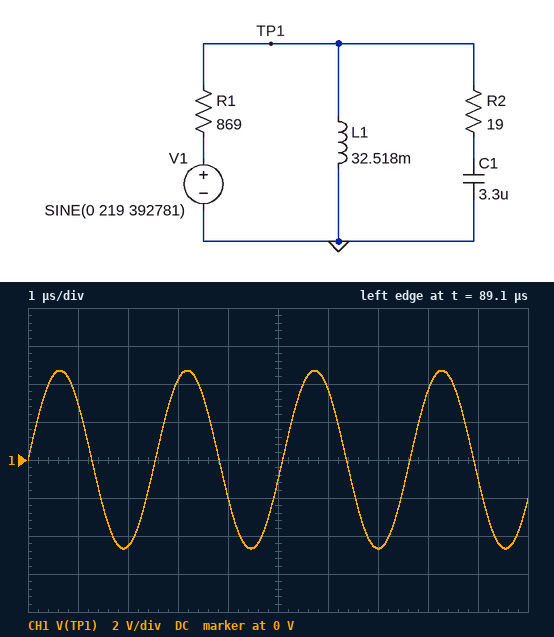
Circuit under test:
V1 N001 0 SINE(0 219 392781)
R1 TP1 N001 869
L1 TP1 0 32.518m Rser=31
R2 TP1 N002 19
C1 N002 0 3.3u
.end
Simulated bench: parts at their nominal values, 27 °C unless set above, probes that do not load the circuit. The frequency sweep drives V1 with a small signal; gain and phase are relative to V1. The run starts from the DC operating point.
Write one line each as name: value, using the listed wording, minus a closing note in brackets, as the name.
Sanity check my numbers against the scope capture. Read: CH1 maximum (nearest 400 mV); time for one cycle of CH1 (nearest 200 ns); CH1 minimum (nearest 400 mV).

CH1 maximum: 4.8 V
time for one cycle of CH1: 2.6 µs
CH1 minimum: -4.8 V
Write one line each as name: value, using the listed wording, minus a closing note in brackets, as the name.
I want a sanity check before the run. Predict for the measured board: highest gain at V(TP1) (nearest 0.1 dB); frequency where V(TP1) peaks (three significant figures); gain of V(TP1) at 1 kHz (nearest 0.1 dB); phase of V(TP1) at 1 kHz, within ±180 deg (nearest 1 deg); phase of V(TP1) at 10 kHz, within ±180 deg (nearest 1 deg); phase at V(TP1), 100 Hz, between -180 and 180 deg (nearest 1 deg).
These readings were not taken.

highest gain at V(TP1): -14.2 dB
frequency where V(TP1) peaks: 487 Hz
gain of V(TP1) at 1 kHz: -22.8 dB
phase of V(TP1) at 1 kHz, within ±180 deg: -56 deg
phase of V(TP1) at 10 kHz, within ±180 deg: -13 deg
phase at V(TP1), 100 Hz, between -180 and 180 deg: 28 deg
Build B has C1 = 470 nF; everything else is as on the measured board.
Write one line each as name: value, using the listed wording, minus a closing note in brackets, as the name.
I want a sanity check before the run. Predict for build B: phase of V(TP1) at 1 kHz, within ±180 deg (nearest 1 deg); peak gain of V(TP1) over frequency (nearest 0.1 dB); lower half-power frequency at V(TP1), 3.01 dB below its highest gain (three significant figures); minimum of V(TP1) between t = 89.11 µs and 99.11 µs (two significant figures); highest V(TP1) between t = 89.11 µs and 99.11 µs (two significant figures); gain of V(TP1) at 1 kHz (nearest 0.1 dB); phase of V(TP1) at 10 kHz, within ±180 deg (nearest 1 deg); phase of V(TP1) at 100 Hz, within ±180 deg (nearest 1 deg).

phase of V(TP1) at 1 kHz, within ±180 deg: 42 deg
peak gain of V(TP1) over frequency: -4.2 dB
lower half-power frequency at V(TP1), 3.01 dB below its highest gain: 1.02 kHz
minimum of V(TP1) between t = 89.11 µs and 99.11 µs: -4.6 V
highest V(TP1) between t = 89.11 µs and 99.11 µs: 4.8 V
gain of V(TP1) at 1 kHz: -7.6 dB
phase of V(TP1) at 10 kHz, within ±180 deg: -58 deg
phase of V(TP1) at 100 Hz, within ±180 deg: 32 deg
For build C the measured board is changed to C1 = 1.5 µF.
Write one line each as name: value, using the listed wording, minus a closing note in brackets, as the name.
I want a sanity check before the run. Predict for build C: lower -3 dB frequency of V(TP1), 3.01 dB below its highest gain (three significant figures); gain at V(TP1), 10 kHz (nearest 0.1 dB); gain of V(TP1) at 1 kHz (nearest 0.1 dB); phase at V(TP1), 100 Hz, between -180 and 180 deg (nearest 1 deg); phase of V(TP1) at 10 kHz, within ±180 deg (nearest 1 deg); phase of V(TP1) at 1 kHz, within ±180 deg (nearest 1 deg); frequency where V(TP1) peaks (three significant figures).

lower -3 dB frequency of V(TP1), 3.01 dB below its highest gain: 564 Hz
gain at V(TP1), 10 kHz: -32.2 dB
gain of V(TP1) at 1 kHz: -13.7 dB
phase at V(TP1), 100 Hz, between -180 and 180 deg: 30 deg
phase of V(TP1) at 10 kHz, within ±180 deg: -28 deg
phase of V(TP1) at 1 kHz, within ±180 deg: -51 deg
frequency where V(TP1) peaks: 724 Hz
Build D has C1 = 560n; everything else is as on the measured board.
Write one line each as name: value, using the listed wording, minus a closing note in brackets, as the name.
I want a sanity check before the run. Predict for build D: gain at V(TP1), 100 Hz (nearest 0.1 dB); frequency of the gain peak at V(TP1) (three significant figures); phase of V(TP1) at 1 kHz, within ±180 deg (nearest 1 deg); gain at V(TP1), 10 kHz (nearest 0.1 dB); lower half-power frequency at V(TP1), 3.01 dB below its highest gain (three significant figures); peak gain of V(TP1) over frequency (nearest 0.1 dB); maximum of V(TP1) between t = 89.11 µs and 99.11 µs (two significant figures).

gain at V(TP1), 100 Hz: -27.6 dB
frequency of the gain peak at V(TP1): 1.19 kHz
phase of V(TP1) at 1 kHz, within ±180 deg: 31 deg
gain at V(TP1), 10 kHz: -28.2 dB
lower half-power frequency at V(TP1), 3.01 dB below its highest gain: 937 Hz
peak gain of V(TP1) over frequency: -4.8 dB
maximum of V(TP1) between t = 89.11 µs and 99.11 µs: 4.8 V
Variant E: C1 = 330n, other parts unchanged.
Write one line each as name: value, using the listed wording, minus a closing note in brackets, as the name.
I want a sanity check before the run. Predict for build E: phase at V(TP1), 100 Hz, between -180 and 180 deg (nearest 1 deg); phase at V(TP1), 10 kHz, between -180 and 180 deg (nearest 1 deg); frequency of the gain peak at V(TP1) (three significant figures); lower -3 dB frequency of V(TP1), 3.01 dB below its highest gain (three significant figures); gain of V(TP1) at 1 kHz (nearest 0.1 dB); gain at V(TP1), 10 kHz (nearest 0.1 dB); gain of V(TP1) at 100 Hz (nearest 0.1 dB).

phase at V(TP1), 100 Hz, between -180 and 180 deg: 32 deg
phase at V(TP1), 10 kHz, between -180 and 180 deg: -65 deg
frequency of the gain peak at V(TP1): 1.55 kHz
lower -3 dB frequency of V(TP1), 3.01 dB below its highest gain: 1.20 kHz
gain of V(TP1) at 1 kHz: -9.3 dB
gain at V(TP1), 10 kHz: -24.5 dB
gain of V(TP1) at 100 Hz: -27.7 dB
